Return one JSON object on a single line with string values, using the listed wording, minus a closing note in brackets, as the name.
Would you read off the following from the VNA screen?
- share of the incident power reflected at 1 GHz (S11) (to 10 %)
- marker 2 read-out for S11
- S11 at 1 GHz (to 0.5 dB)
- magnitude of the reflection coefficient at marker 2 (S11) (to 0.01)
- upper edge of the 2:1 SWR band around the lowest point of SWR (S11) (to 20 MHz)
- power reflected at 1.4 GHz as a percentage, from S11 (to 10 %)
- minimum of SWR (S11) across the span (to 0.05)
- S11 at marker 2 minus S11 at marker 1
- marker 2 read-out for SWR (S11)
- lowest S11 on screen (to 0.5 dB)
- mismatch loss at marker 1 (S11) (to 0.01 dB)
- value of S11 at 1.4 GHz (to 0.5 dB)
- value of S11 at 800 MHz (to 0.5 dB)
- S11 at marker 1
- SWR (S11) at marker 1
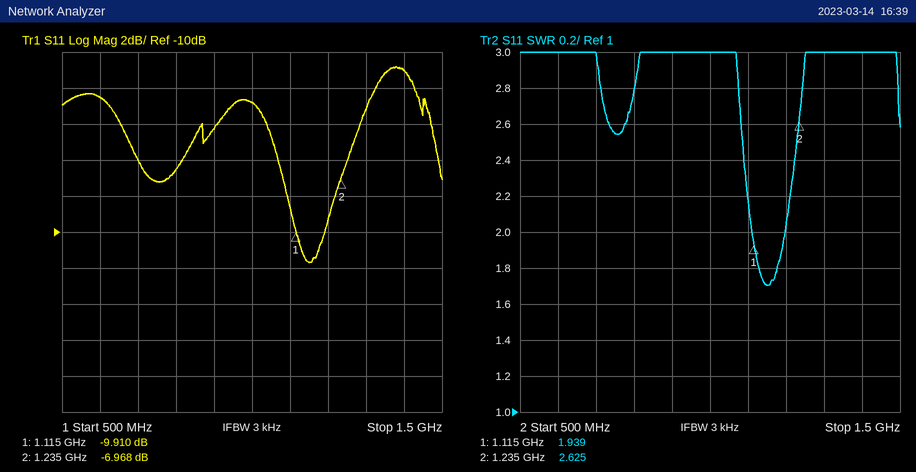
{"share of the incident power reflected at 1 GHz (S11)": "50 %", "marker 2 read-out for S11": "-6.968 dB", "S11 at 1 GHz": "-3.0 dB", "magnitude of the reflection coefficient at marker 2 (S11)": "0.45", "upper edge of the 2:1 SWR band around the lowest point of SWR (S11)": "1.20 GHz", "power reflected at 1.4 GHz as a percentage, from S11": "80 %", "minimum of SWR (S11) across the span": "1.70", "S11 at marker 2 minus S11 at marker 1": "2.942 dB", "marker 2 read-out for SWR": "2.625", "lowest S11 on screen": "-11.5 dB", "mismatch loss at marker 1 (S11)": "0.47 dB", "value of S11 at 1.4 GHz": "-1.0 dB", "value of S11 at 800 MHz": "-6.5 dB", "S11 at marker 1": "-9.910 dB", "SWR (S11) at marker 1": "1.939"}
